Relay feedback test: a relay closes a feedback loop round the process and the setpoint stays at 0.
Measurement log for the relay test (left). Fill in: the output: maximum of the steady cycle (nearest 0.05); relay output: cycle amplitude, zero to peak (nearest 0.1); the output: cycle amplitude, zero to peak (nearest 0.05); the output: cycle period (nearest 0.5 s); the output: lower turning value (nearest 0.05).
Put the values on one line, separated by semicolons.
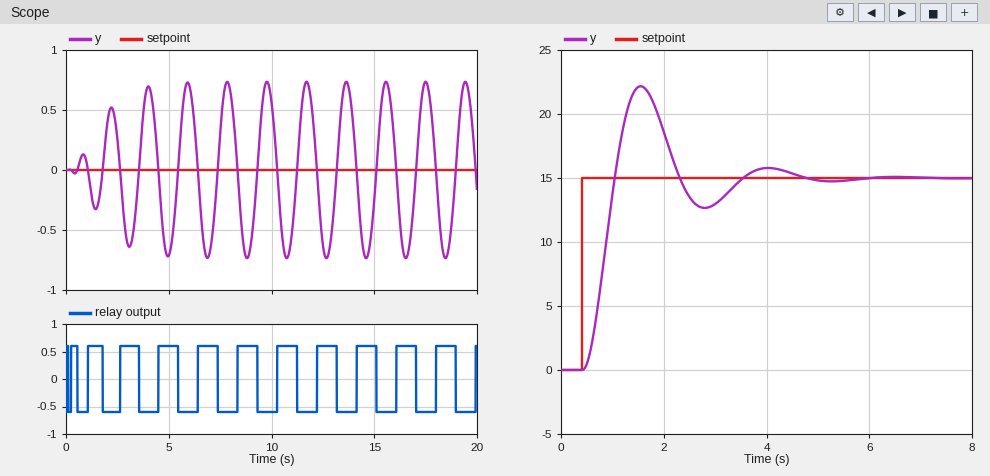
0.75; 0.6; 0.75; 2.0 s; -0.75
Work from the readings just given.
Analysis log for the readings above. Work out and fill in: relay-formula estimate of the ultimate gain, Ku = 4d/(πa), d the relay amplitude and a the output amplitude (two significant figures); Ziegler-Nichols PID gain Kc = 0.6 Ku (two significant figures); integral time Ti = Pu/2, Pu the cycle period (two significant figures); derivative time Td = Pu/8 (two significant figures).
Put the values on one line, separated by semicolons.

1.0; 0.60; 1.0 s; 0.25 s
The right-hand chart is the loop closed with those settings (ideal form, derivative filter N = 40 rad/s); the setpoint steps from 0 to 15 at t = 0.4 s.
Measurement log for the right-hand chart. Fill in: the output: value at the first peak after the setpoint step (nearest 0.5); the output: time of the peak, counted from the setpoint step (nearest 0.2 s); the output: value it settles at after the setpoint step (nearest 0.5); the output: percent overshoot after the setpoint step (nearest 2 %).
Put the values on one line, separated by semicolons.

22.0; 1.2 s; 15.0; 48 %
